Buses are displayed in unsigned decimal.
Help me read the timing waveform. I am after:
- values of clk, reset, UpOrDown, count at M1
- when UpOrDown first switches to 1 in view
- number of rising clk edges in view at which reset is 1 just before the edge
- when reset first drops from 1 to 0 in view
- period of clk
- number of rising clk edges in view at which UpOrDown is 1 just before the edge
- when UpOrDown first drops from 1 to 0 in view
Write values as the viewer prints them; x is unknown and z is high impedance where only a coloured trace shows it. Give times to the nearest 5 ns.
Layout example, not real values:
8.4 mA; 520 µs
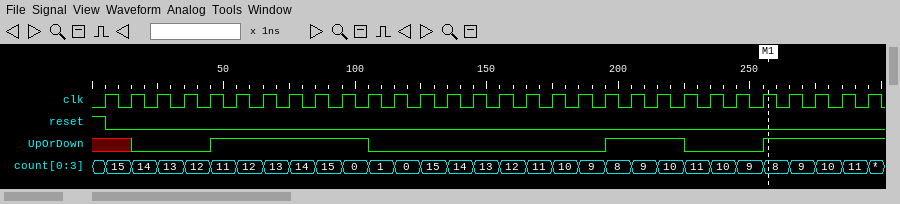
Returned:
clk=1, reset=0, UpOrDown=1, count=8; 45 ns; 1; 5 ns; 10 ns; 13; 105 ns
